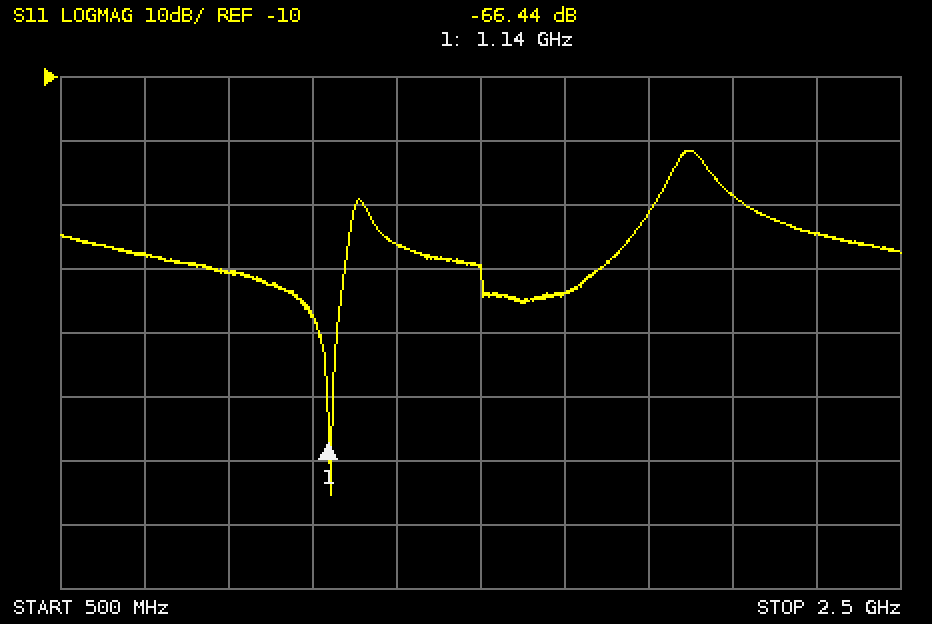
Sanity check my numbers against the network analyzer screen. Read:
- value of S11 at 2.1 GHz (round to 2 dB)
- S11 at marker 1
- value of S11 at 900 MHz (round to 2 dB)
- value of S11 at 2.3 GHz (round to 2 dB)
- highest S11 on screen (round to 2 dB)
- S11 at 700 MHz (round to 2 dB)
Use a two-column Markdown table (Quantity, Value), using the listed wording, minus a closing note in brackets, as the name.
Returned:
| Quantity | Value |
|---|---|
| value of S11 at 2.1 GHz | -28 dB |
| S11 at marker 1 | -66.44 dB |
| value of S11 at 900 MHz | -40 dB |
| value of S11 at 2.3 GHz | -34 dB |
| highest S11 on screen | -22 dB |
| S11 at 700 MHz | -38 dB |
